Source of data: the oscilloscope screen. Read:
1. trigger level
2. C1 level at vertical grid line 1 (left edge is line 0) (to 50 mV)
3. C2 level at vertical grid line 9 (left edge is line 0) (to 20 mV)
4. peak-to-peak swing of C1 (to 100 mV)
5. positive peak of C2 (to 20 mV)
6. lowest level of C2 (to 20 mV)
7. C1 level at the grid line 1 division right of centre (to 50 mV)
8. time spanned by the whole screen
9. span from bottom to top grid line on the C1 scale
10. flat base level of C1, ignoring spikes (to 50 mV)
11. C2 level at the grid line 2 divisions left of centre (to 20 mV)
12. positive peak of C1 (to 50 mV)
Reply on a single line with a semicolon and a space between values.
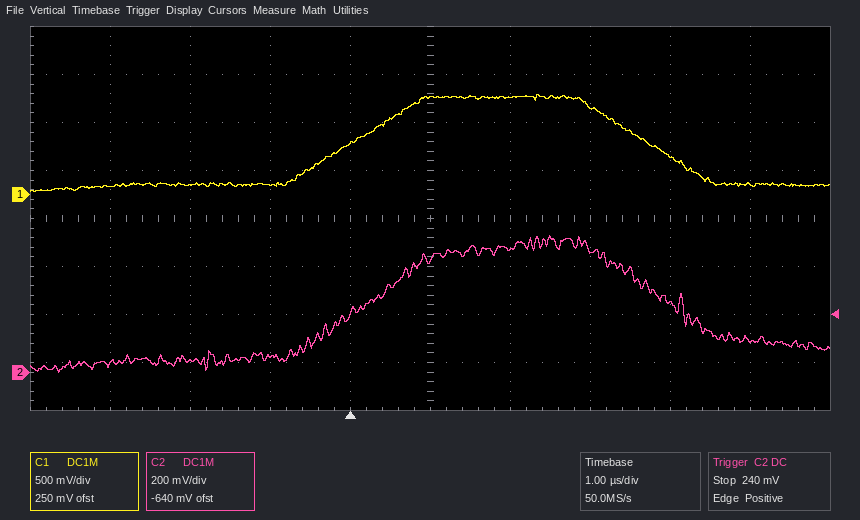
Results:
240 mV; 100 mV; 140 mV; 1.00 V; 560 mV; 0 mV; 1.00 V; 10 µs; 4 V; 100 mV; 60 mV; 1.05 V
